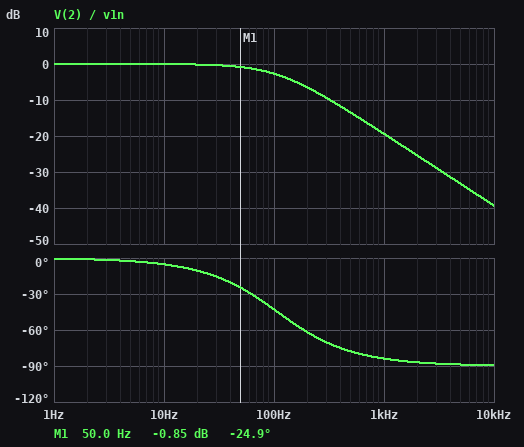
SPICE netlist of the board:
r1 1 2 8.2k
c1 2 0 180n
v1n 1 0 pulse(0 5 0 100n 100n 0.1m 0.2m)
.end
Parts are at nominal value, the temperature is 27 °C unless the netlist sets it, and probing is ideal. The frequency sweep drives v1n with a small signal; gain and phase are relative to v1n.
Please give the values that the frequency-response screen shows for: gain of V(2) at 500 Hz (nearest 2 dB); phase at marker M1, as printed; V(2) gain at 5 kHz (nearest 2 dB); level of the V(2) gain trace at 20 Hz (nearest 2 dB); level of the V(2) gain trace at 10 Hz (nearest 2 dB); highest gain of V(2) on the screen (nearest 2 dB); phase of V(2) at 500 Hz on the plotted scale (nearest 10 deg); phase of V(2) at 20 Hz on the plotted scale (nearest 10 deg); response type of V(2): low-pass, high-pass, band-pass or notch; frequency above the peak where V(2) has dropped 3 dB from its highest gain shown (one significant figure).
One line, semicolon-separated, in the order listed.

-14 dB; -24.9 deg; -34 dB; 0 dB; 0 dB; 0 dB; -80 deg; -10 deg; low-pass; 100 Hz
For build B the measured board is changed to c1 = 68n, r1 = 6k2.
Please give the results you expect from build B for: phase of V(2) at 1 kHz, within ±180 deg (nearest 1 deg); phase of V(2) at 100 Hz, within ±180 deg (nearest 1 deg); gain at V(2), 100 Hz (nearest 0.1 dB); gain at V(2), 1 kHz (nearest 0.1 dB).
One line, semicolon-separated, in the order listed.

-69 deg; -15 deg; -0.3 dB; -9.0 dB
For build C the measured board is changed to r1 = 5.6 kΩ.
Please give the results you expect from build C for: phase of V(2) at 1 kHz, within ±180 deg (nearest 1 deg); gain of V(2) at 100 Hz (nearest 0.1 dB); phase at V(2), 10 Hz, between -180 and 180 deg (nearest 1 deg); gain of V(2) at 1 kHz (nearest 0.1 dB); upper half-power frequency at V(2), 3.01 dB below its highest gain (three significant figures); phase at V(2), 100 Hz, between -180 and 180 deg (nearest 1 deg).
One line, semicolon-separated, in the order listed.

-81 deg; -1.5 dB; -4 deg; -16.1 dB; 158 Hz; -32 deg
